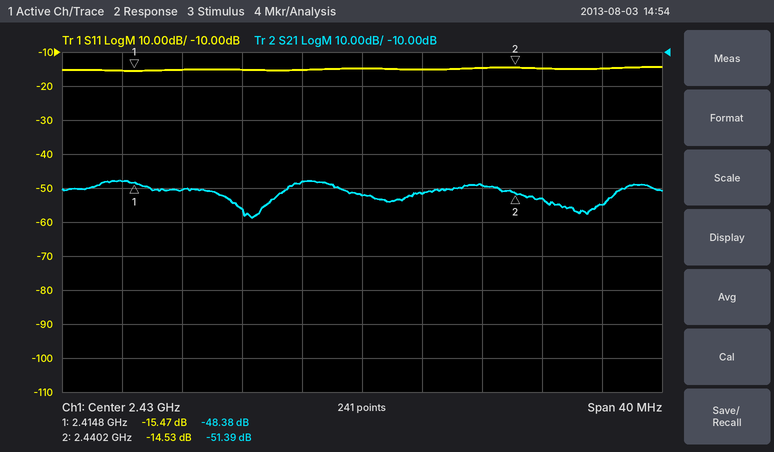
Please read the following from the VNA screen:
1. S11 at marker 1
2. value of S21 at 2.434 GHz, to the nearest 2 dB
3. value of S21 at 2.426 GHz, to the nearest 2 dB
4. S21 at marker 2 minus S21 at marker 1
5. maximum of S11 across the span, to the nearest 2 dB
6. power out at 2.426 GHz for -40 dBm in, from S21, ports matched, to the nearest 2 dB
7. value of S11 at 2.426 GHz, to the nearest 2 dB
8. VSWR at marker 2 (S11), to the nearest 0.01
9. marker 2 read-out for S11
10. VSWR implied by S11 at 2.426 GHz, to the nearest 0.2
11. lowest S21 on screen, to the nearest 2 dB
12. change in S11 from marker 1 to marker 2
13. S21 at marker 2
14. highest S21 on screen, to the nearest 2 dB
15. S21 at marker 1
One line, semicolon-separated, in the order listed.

-15.47 dB; -52 dB; -48 dB; -3.01 dB; -14 dB; -88 dBm; -16 dB; 1.46; -14.53 dB; 1.4; -58 dB; 0.94 dB; -51.39 dB; -48 dB; -48.38 dB
